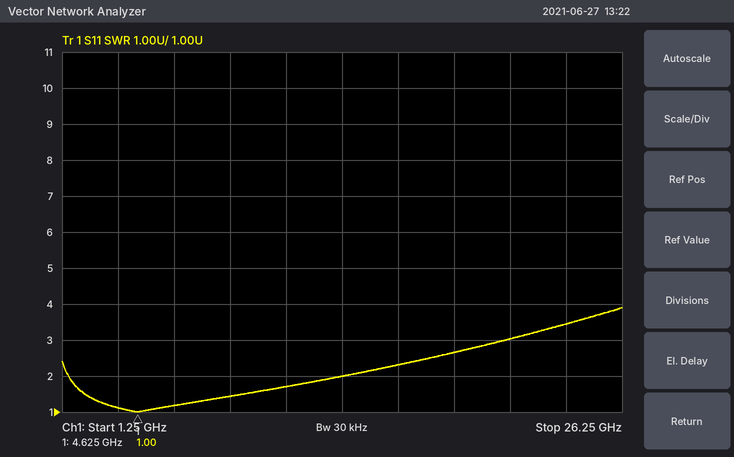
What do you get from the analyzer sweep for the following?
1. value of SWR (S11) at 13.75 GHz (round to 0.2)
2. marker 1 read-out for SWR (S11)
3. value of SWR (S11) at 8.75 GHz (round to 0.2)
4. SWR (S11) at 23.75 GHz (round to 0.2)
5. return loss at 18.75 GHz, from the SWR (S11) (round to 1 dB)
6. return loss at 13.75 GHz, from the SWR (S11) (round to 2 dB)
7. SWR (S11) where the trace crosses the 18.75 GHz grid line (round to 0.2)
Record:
2.0
1.00
1.4
3.4
7 dB
10 dB
2.6
